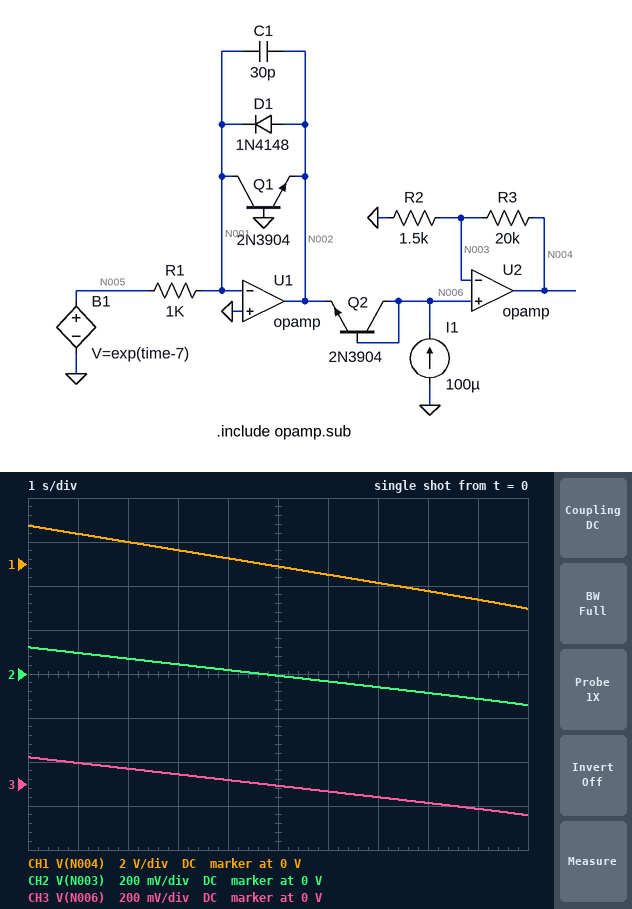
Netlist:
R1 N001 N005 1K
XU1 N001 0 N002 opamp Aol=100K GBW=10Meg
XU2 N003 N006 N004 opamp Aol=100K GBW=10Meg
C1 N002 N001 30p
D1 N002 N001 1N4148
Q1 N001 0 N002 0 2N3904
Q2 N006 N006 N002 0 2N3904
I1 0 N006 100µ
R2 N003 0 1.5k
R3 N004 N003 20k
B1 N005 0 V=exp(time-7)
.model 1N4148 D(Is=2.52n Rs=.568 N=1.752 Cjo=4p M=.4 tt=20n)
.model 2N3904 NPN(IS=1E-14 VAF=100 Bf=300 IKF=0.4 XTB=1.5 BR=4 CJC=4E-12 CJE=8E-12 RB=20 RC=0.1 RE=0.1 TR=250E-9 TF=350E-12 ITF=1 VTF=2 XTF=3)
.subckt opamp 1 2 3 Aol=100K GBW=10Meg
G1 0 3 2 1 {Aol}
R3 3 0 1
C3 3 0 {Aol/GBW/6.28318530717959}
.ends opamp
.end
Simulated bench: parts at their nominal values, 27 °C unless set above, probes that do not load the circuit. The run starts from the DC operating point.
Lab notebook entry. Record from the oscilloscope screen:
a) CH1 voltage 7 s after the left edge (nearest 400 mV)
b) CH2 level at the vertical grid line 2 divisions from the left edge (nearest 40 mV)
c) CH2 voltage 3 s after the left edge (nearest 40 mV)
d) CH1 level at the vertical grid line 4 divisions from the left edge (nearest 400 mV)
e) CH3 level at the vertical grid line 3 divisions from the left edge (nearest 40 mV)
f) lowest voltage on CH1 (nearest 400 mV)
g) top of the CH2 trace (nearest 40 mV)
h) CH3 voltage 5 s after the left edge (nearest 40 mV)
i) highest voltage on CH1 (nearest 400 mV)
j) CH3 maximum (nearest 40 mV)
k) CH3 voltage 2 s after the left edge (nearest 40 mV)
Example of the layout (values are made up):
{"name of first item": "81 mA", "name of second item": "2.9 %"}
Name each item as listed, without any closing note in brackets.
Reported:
{"CH1 voltage 7 s after the left edge": "-800 mV", "CH2 level at the vertical grid line 2 divisions from the left edge": "80 mV", "CH2 voltage 3 s after the left edge": "40 mV", "CH1 level at the vertical grid line 4 divisions from the left edge": "400 mV", "CH3 level at the vertical grid line 3 divisions from the left edge": "40 mV", "lowest voltage on CH1": "-2.0 V", "top of the CH2 trace": "120 mV", "CH3 voltage 5 s after the left edge": "0 V", "highest voltage on CH1": "1.6 V", "CH3 maximum": "120 mV", "CH3 voltage 2 s after the left edge": "80 mV"}
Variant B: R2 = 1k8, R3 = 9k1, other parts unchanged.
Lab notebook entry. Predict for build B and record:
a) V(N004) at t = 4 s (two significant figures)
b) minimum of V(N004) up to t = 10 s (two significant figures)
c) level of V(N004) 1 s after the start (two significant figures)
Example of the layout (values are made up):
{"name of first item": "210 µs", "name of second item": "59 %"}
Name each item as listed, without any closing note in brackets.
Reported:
{"V(N004) at t = 4 s": "110 mV", "minimum of V(N004) up to t = 10 s": "-860 mV", "level of V(N004) 1 s after the start": "580 mV"}
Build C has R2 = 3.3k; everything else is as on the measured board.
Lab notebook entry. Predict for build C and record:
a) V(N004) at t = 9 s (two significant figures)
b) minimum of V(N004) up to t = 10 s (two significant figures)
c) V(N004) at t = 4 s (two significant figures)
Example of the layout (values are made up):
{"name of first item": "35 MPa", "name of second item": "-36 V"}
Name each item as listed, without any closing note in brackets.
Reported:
{"V(N004) at t = 9 s": "-800 mV", "minimum of V(N004) up to t = 10 s": "-1.0 V", "V(N004) at t = 4 s": "130 mV"}
